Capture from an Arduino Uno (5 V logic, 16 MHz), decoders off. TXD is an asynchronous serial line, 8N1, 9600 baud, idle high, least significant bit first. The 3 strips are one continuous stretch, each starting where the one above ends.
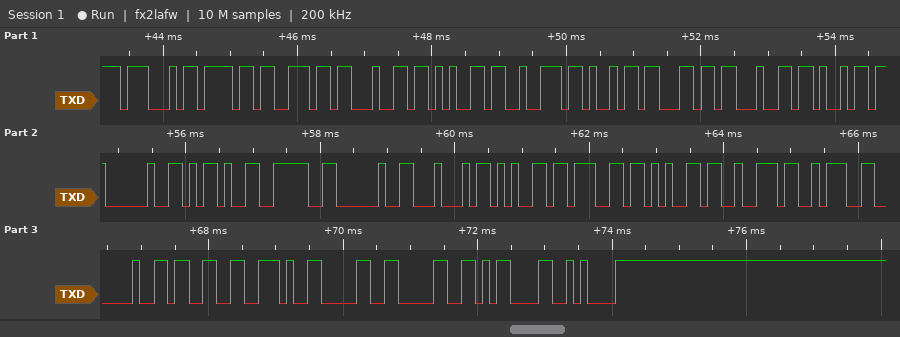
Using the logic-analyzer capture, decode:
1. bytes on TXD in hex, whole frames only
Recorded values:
47 6F 6E 64 65 72 69 6C 64 69 20 2D 3E 20 44 65 67 65 72 3A 20 33 2E 30 30 0D 0A
